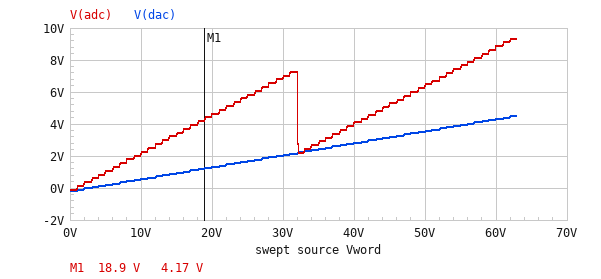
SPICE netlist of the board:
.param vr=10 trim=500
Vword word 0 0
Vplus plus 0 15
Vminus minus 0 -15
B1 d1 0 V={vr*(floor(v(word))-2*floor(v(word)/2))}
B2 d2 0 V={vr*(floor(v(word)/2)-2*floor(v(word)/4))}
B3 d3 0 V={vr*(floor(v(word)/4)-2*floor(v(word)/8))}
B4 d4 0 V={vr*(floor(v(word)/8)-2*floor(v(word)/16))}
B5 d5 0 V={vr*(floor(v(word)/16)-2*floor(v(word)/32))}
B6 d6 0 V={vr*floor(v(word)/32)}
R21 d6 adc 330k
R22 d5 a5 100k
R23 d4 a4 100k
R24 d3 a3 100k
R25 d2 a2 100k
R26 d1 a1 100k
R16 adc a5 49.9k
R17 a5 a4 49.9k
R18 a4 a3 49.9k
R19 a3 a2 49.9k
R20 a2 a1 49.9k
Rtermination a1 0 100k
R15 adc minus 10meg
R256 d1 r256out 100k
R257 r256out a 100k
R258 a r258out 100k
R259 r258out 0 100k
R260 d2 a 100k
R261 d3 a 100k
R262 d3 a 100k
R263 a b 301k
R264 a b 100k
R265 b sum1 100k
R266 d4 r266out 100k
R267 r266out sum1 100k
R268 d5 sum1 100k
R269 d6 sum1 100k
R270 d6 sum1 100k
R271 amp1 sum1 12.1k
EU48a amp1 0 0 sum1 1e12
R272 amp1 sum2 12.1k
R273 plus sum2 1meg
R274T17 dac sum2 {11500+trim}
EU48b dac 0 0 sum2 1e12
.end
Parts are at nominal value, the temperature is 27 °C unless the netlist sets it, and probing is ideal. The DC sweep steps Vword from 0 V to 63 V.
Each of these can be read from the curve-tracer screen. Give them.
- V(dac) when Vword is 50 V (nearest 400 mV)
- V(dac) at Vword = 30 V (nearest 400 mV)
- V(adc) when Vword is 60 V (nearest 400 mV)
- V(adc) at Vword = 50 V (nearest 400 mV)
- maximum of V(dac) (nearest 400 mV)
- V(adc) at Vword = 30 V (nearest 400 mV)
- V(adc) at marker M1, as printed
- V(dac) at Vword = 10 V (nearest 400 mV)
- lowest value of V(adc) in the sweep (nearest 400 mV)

3.6 V
2.0 V
8.8 V
6.4 V
4.4 V
6.8 V
4.17 V
400 mV
0 V
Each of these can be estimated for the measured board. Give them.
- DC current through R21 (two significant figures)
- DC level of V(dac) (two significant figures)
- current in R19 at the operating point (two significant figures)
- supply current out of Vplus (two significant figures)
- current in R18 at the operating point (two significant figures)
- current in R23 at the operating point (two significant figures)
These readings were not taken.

350 nA
-180 mV
140 nA
15 µA
290 nA
290 nA
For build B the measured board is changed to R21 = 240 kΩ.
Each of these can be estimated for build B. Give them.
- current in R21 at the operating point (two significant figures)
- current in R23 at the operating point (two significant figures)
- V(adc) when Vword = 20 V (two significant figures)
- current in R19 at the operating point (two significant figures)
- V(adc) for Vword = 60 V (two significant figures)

440 nA
260 nA
4.3 V
130 nA
8.9 V
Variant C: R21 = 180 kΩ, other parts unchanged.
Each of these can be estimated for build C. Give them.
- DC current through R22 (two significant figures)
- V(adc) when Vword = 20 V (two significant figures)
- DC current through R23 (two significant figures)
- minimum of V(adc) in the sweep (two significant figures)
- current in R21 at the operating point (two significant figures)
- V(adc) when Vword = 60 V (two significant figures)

480 nA
3.9 V
240 nA
-96 mV
530 nA
9.0 V
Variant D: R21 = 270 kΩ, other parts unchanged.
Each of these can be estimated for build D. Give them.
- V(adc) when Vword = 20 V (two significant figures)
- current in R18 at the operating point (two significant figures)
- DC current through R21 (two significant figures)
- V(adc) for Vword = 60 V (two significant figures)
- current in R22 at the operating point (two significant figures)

4.4 V
270 nA
400 nA
8.9 V
540 nA
